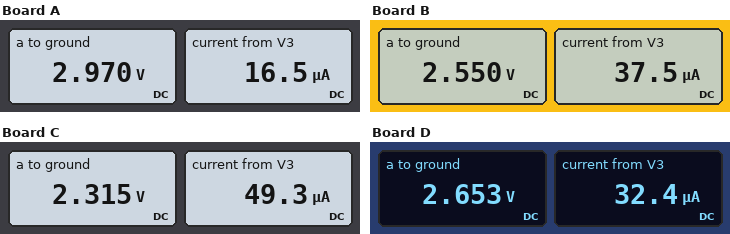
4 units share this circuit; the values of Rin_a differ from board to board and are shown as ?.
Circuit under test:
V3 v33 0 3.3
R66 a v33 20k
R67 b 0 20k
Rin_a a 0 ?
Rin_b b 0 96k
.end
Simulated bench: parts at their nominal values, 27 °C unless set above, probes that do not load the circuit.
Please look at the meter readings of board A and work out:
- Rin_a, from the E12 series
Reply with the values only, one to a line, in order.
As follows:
180 kΩ
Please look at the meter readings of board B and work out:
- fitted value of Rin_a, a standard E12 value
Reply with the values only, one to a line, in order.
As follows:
68 kΩ
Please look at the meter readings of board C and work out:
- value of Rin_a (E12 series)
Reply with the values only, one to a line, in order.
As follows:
47 kΩ
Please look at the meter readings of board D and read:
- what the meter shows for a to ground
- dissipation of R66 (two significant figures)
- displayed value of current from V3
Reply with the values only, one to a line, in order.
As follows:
2.653 V
21 µW
32.4 µA
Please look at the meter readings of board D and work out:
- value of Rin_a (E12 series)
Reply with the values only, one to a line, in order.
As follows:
82 kΩ
